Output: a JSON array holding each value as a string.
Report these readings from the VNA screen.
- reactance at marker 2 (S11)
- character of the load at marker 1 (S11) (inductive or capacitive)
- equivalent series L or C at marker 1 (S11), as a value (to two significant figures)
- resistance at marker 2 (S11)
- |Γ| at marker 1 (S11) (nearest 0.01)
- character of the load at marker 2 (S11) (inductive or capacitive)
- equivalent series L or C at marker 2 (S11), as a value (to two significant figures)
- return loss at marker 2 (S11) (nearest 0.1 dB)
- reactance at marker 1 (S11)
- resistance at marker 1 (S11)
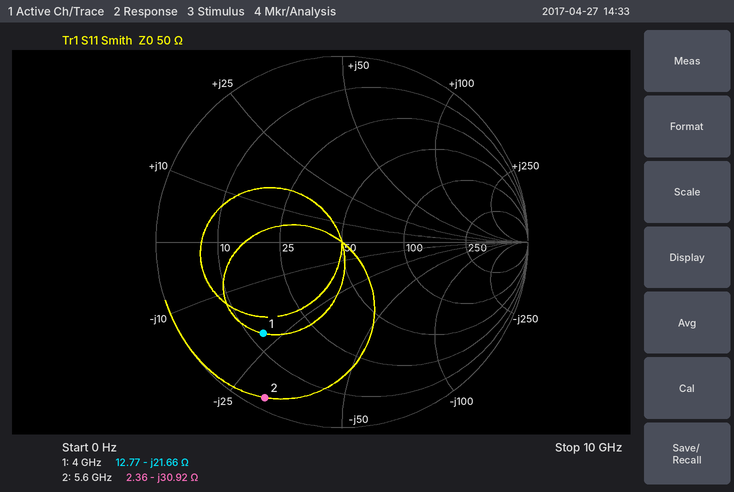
["-30.92 Ω", "capacitive", "1.8 pF", "2.36 Ω", "0.65", "capacitive", "920 fF", "0.6 dB", "-21.66 Ω", "12.77 Ω"]
